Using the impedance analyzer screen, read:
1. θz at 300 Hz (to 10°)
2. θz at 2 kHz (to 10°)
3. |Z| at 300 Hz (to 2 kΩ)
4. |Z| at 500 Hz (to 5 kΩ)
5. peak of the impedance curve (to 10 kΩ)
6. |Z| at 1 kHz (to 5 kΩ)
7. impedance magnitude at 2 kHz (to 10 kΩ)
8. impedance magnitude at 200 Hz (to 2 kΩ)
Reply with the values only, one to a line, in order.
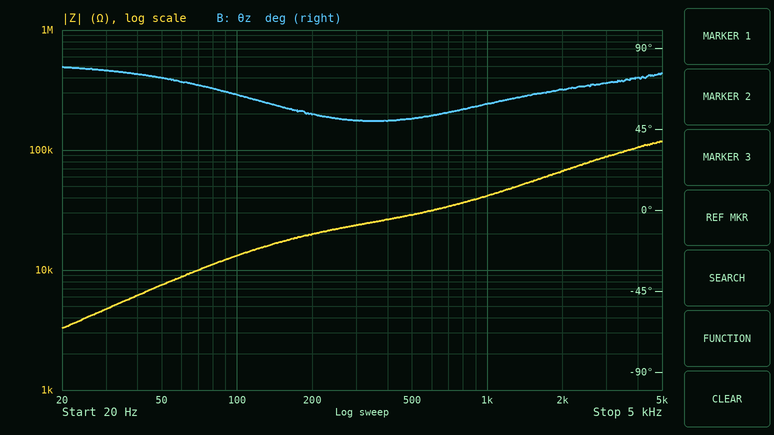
50°
70°
24 kΩ
30 kΩ
120 kΩ
40 kΩ
70 kΩ
20 kΩ
